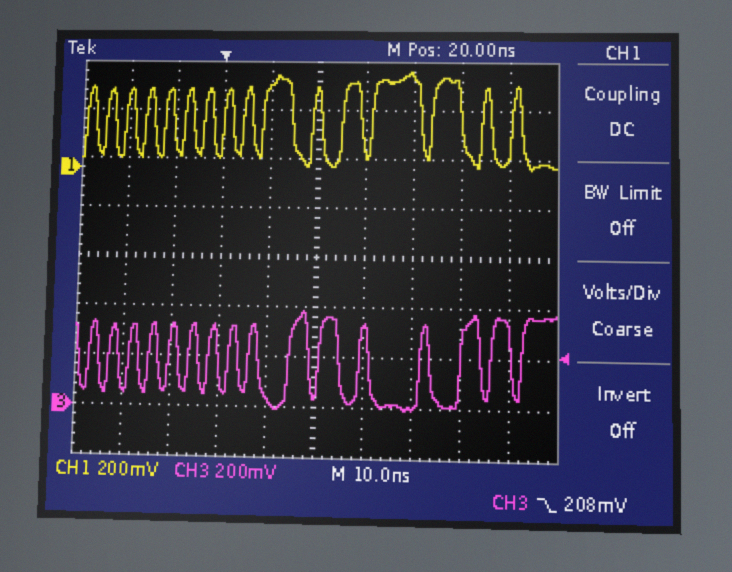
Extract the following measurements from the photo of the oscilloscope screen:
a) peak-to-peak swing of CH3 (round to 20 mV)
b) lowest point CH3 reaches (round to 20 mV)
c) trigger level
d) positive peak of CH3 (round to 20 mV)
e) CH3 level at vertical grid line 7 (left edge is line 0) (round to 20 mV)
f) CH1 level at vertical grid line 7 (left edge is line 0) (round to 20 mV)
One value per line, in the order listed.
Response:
380 mV
0 mV
208 mV
380 mV
0 mV
380 mV
